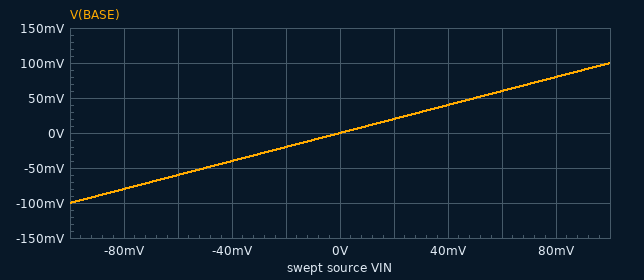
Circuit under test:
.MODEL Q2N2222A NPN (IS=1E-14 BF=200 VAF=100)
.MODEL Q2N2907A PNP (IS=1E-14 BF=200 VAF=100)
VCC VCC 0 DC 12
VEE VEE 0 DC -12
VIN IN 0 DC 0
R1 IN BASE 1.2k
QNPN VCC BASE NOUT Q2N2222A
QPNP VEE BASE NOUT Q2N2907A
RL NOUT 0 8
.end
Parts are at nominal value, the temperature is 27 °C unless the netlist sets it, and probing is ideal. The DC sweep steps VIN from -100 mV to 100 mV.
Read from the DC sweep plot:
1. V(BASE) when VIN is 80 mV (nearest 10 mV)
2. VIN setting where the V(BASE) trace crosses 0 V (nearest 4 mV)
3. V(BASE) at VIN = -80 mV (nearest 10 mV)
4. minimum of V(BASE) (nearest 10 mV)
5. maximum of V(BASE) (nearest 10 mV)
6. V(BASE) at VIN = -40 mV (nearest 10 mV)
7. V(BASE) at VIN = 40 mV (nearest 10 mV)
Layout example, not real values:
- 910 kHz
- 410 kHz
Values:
- 80 mV
- 0 V
- -80 mV
- -100 mV
- 100 mV
- -40 mV
- 40 mV
